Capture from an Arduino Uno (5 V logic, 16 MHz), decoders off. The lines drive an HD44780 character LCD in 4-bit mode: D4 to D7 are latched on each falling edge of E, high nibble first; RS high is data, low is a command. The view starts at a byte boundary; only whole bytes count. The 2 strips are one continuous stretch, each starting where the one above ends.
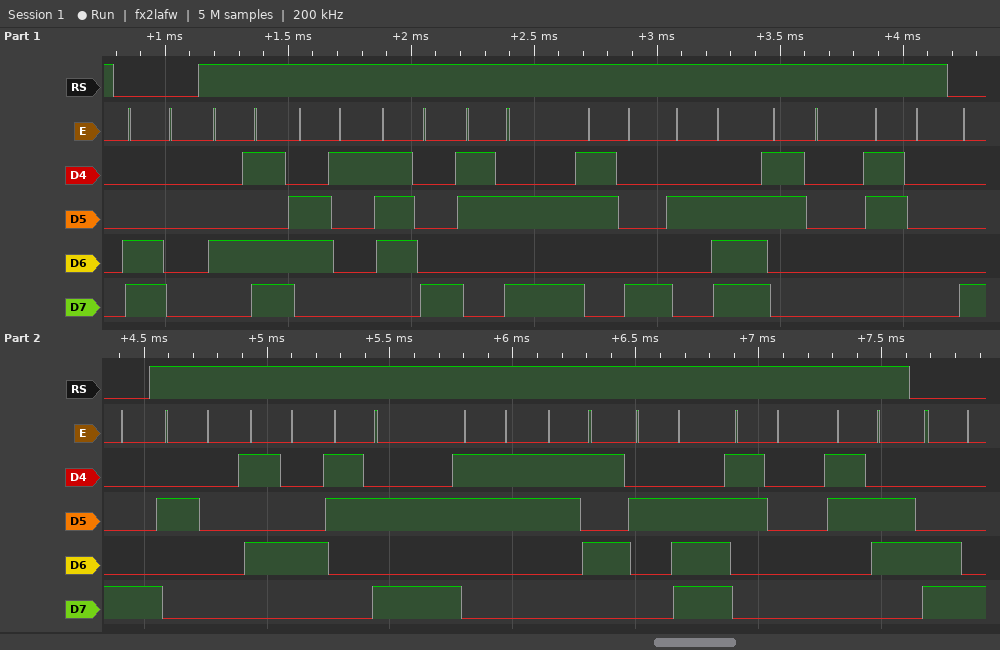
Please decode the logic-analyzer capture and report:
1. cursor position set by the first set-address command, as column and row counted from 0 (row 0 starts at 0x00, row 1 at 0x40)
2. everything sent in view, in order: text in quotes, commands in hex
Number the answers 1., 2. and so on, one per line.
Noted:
1. column 0, row 1
2. 0xC0 "Max:8.00" 0x88 " T:35.06" 0xC8
